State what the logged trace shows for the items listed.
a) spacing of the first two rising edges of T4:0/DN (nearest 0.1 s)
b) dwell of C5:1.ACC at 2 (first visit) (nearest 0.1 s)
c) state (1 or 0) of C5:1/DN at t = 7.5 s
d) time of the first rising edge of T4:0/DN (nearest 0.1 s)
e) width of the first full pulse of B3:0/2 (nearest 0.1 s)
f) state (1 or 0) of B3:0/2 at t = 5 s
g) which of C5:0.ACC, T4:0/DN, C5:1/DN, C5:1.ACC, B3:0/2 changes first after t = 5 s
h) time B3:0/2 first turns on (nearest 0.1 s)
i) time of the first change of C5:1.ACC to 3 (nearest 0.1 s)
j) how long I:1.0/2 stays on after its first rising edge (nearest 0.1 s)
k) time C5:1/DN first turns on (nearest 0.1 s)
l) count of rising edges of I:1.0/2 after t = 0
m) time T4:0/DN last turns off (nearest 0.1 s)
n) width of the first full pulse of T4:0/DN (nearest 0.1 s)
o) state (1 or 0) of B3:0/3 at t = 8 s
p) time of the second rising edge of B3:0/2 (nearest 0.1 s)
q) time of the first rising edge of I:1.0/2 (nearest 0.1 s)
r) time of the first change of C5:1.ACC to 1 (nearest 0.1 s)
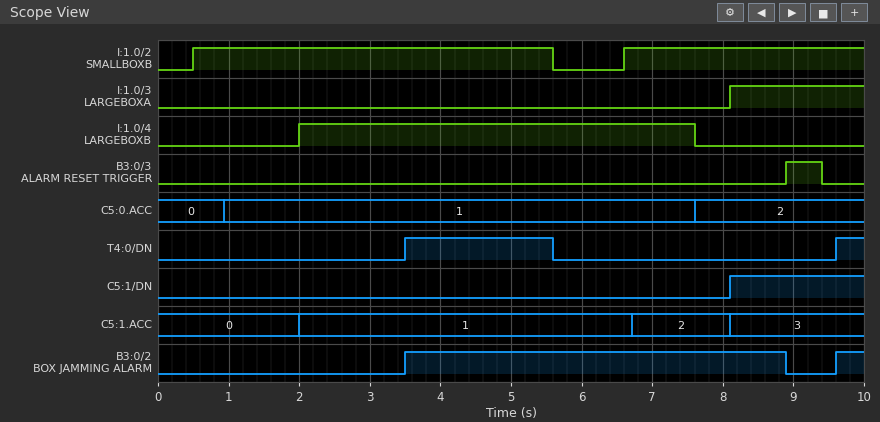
6.1 s
1.4 s
0
3.5 s
5.4 s
1
T4:0/DN
3.5 s
8.1 s
5.1 s
8.1 s
2
5.6 s
2.1 s
0
9.6 s
0.5 s
2.0 s
